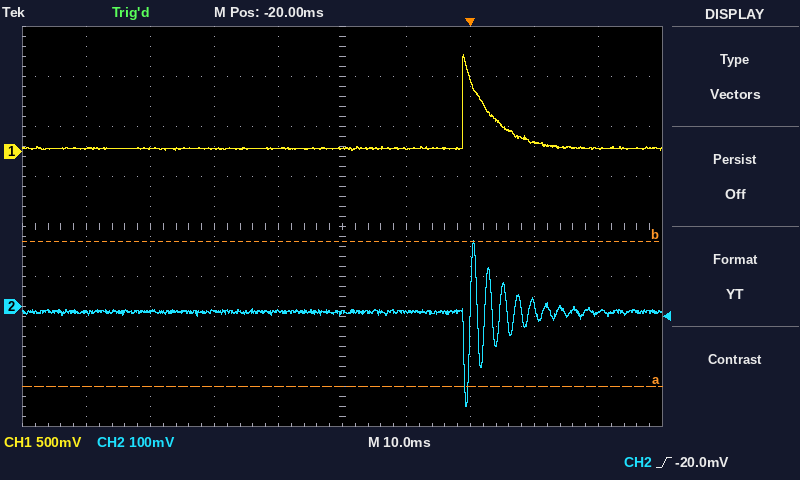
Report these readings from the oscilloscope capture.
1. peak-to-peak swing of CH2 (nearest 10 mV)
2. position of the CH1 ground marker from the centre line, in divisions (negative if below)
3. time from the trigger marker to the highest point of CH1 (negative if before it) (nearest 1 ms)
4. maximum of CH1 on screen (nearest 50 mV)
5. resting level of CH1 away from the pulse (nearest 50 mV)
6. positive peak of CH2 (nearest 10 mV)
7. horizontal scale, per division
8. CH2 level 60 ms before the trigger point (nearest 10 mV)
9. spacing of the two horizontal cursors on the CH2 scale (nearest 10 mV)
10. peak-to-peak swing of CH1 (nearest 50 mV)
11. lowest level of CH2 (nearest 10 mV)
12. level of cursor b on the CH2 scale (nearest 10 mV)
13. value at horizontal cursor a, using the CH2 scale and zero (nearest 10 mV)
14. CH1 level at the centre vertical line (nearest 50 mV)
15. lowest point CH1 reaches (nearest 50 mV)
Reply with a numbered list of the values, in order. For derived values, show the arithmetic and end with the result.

1. 130 mV − (-200 mV) = 330 mV
2. +1.5 div
3. -1 ms
4. 950 mV
5. 50 mV
6. 130 mV
7. 10 ms
8. -10 mV
9. 290 mV
10. 950 mV − (0 mV) = 950 mV
11. -200 mV
12. 130 mV
13. -160 mV
14. 50 mV
15. 0 mV
